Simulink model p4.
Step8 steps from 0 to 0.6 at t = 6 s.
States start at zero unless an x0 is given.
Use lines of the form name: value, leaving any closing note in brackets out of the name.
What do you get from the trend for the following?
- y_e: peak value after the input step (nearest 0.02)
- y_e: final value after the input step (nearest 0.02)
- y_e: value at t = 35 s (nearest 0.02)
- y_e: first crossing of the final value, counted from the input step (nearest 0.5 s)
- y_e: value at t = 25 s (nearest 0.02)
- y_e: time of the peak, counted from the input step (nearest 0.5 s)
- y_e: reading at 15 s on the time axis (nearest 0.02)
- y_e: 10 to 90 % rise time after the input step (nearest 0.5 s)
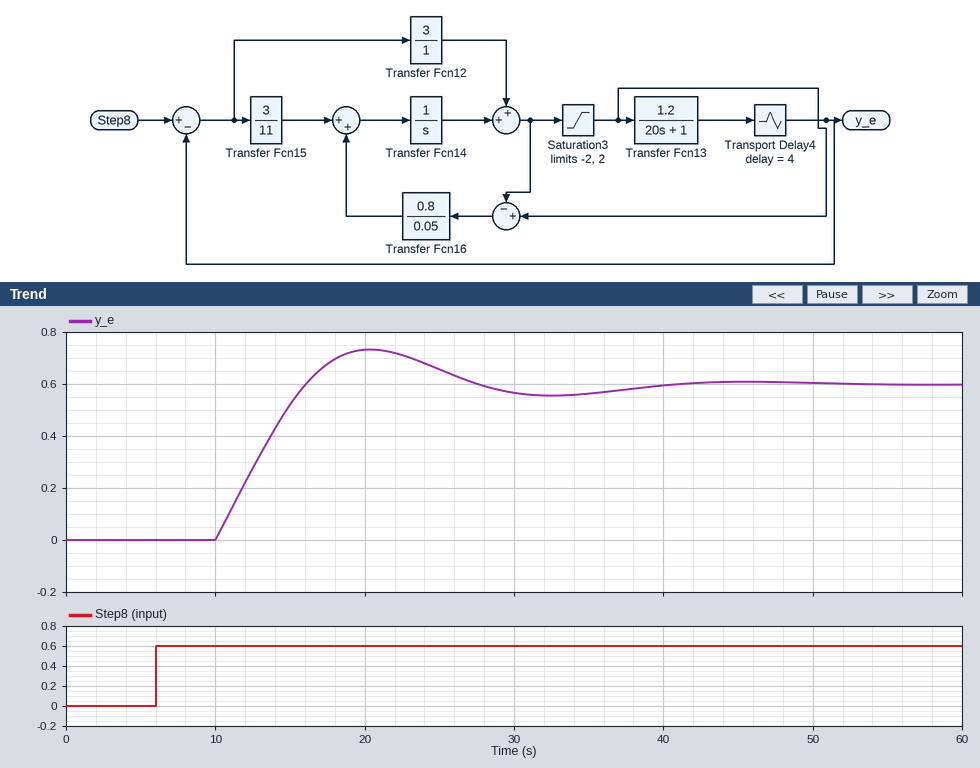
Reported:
y_e: peak value after the input step: 0.74
y_e: final value after the input step: 0.60
y_e: value at t = 35 s: 0.56
y_e: first crossing of the final value, counted from the input step: 10.0 s
y_e: value at t = 25 s: 0.66
y_e: time of the peak, counted from the input step: 14.5 s
y_e: reading at 15 s on the time axis: 0.52
y_e: 10 to 90 % rise time after the input step: 4.5 s
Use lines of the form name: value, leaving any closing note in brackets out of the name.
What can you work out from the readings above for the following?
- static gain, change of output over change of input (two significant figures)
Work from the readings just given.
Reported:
static gain, change of output over change of input: 1.0
